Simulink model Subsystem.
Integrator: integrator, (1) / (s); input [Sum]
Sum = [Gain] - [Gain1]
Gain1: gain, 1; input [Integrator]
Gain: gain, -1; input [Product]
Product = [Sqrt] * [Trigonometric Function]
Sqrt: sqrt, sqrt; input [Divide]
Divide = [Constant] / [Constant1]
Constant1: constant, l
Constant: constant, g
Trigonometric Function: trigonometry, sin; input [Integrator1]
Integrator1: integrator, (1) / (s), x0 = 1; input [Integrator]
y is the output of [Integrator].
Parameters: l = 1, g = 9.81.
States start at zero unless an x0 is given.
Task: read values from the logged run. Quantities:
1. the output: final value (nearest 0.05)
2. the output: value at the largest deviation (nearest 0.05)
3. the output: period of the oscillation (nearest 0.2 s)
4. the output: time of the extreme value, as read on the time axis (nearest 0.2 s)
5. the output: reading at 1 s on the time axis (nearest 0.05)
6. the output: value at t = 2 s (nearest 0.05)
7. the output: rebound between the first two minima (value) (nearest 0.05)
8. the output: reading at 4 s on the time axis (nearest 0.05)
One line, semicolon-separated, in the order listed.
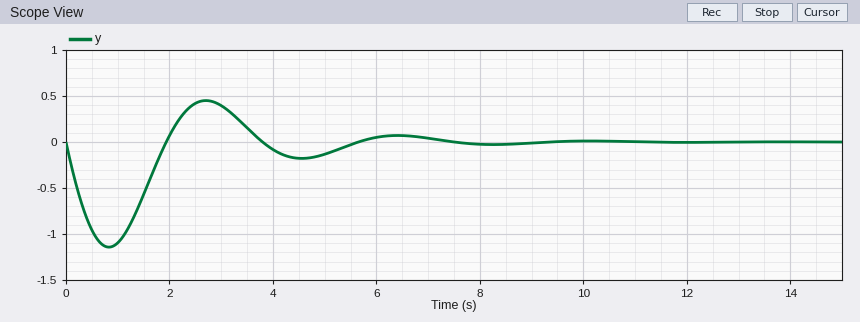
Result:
0.00; -1.15; 3.8 s; 0.8 s; -1.10; 0.05; 0.45; -0.10
